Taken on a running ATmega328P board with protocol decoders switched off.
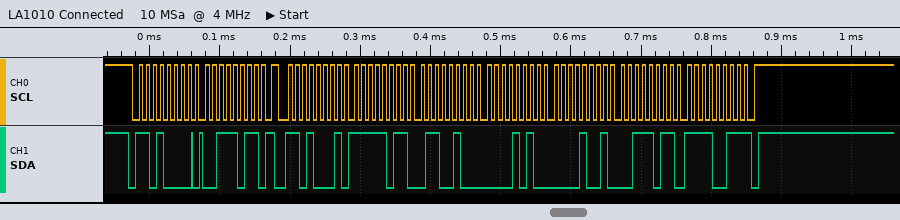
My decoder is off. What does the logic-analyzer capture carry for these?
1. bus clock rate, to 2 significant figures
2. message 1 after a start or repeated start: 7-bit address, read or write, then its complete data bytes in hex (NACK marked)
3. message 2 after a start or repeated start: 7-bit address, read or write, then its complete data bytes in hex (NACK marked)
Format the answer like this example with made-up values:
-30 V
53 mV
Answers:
100 kHz
0x68 write: 3B
0x68 read: FB 64 0A 09 3B F3 NACK
